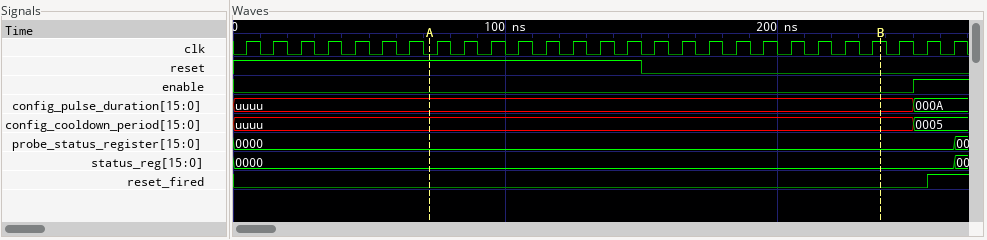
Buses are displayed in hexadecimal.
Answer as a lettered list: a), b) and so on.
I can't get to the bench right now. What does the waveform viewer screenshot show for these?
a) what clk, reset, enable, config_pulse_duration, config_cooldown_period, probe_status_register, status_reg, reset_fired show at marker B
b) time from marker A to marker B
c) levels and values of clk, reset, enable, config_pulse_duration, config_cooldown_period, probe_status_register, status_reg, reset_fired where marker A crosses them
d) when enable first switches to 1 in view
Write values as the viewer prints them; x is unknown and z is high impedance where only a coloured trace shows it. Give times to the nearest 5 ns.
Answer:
a) clk=1, reset=0, enable=0, config_pulse_duration=uuuu, config_cooldown_period=uuuu, probe_status_register=0000, status_reg=0000, reset_fired=0
b) 165 ns
c) clk=0, reset=1, enable=0, config_pulse_duration=uuuu, config_cooldown_period=uuuu, probe_status_register=0000, status_reg=0000, reset_fired=0
d) 250 ns
